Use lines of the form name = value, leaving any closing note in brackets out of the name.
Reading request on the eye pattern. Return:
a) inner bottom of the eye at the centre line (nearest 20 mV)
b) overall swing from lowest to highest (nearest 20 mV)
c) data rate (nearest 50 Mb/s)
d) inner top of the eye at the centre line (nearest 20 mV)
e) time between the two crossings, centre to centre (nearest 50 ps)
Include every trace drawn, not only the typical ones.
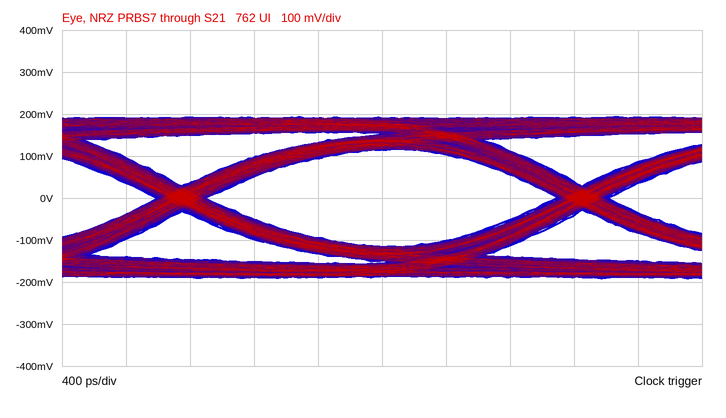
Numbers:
inner bottom of the eye at the centre line = -120 mV
overall swing from lowest to highest = 380 mV
data rate = 400 Mb/s
inner top of the eye at the centre line = 120 mV
time between the two crossings, centre to centre = 2.50 ns
